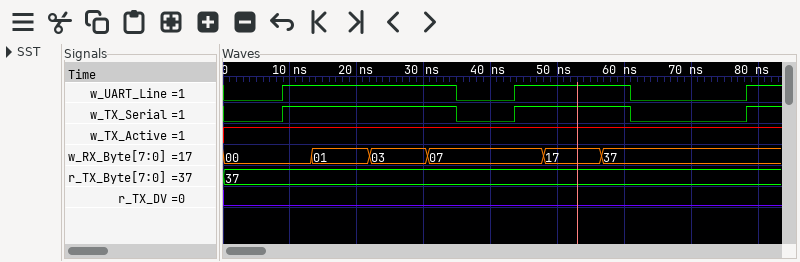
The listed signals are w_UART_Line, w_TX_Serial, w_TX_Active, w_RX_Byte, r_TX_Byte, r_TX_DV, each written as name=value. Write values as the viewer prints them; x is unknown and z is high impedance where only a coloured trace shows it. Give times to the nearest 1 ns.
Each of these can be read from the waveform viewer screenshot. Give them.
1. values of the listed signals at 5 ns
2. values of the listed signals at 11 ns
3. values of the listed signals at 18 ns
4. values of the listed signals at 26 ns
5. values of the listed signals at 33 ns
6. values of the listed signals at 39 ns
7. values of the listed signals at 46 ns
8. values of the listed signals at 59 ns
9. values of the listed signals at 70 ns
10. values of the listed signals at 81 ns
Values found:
w_UART_Line=0, w_TX_Serial=0, w_TX_Active=1, w_RX_Byte=00, r_TX_Byte=37, r_TX_DV=0
w_UART_Line=1, w_TX_Serial=1, w_TX_Active=1, w_RX_Byte=00, r_TX_Byte=37, r_TX_DV=0
w_UART_Line=1, w_TX_Serial=1, w_TX_Active=1, w_RX_Byte=01, r_TX_Byte=37, r_TX_DV=0
w_UART_Line=1, w_TX_Serial=1, w_TX_Active=1, w_RX_Byte=03, r_TX_Byte=37, r_TX_DV=0
w_UART_Line=1, w_TX_Serial=1, w_TX_Active=1, w_RX_Byte=07, r_TX_Byte=37, r_TX_DV=0
w_UART_Line=0, w_TX_Serial=0, w_TX_Active=1, w_RX_Byte=07, r_TX_Byte=37, r_TX_DV=0
w_UART_Line=1, w_TX_Serial=1, w_TX_Active=1, w_RX_Byte=07, r_TX_Byte=37, r_TX_DV=0
w_UART_Line=1, w_TX_Serial=1, w_TX_Active=1, w_RX_Byte=37, r_TX_Byte=37, r_TX_DV=0
w_UART_Line=0, w_TX_Serial=0, w_TX_Active=1, w_RX_Byte=37, r_TX_Byte=37, r_TX_DV=0
w_UART_Line=1, w_TX_Serial=1, w_TX_Active=1, w_RX_Byte=37, r_TX_Byte=37, r_TX_DV=0
